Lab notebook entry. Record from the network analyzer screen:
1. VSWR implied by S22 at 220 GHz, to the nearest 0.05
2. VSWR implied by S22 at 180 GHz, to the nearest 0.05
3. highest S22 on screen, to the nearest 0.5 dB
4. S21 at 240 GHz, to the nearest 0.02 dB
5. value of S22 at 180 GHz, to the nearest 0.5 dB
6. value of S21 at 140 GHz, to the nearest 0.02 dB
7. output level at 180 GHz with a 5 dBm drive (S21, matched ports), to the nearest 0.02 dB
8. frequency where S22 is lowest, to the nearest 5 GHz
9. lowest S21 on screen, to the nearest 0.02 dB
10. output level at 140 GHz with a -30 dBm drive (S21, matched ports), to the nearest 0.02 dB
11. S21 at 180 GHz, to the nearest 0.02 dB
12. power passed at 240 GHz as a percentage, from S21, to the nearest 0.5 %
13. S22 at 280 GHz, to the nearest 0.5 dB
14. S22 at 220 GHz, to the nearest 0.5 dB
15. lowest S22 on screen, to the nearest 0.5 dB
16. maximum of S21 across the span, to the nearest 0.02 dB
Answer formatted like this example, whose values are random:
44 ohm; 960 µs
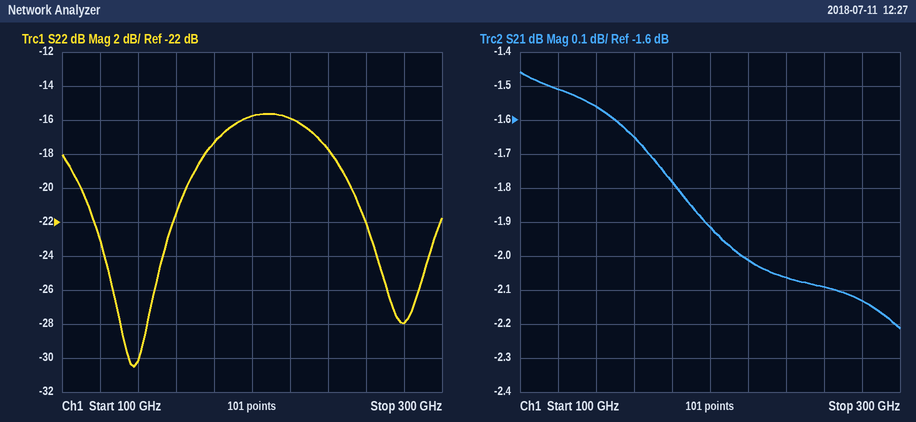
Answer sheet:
1.40; 1.30; -15.5 dB; -2.06 dB; -17.5 dB; -1.56 dB; 3.22 dBm; 140 GHz; -2.22 dB; -31.56 dBm; -1.78 dB; 62.0 %; -28.0 dB; -16.0 dB; -30.5 dB; -1.46 dB
